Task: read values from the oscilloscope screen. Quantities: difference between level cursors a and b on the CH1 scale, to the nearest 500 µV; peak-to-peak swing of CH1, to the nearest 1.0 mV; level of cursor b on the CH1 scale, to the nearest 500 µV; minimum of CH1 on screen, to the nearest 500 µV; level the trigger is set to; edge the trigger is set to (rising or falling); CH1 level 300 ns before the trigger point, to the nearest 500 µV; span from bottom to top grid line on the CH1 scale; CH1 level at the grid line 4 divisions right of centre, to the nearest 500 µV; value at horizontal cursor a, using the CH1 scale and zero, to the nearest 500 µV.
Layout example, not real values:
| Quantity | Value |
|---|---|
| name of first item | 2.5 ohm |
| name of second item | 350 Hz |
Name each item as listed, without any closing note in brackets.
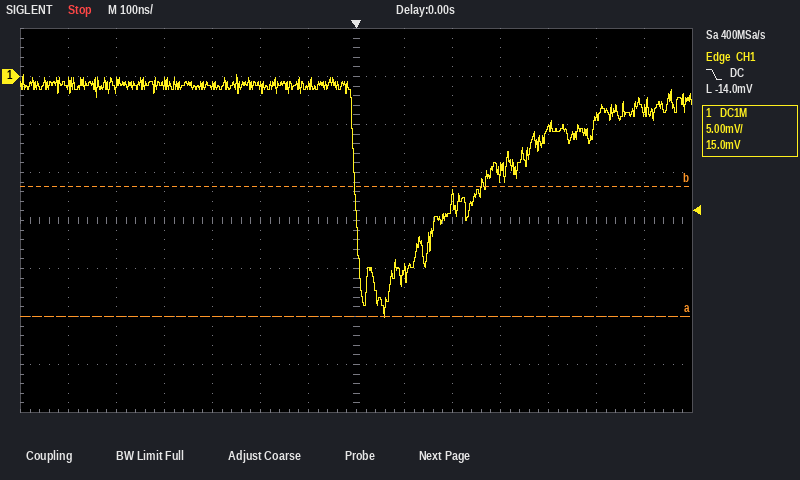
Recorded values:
| Quantity | Value |
|---|---|
| difference between level cursors a and b on the CH1 scale, to the nearest 500 µV | 13.5 mV |
| peak-to-peak swing of CH1, to the nearest 1.0 mV | 25.0 mV |
| level of cursor b on the CH1 scale, to the nearest 500 µV | -11.5 mV |
| minimum of CH1 on screen, to the nearest 500 µV | -25.0 mV |
| level the trigger is set to | -14.0 mV |
| edge the trigger is set to | falling |
| CH1 level 300 ns before the trigger point, to the nearest 500 µV | -1.0 mV |
| span from bottom to top grid line on the CH1 scale | 40 mV |
| CH1 level at the grid line 4 divisions right of centre, to the nearest 500 µV | -5.5 mV |
| value at horizontal cursor a, using the CH1 scale and zero, to the nearest 500 µV | -25.0 mV |
